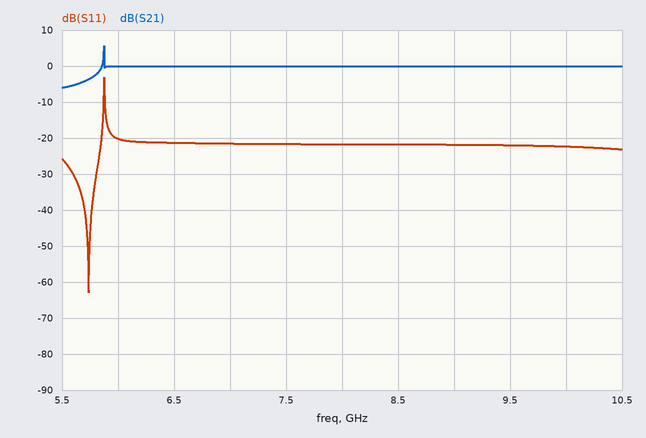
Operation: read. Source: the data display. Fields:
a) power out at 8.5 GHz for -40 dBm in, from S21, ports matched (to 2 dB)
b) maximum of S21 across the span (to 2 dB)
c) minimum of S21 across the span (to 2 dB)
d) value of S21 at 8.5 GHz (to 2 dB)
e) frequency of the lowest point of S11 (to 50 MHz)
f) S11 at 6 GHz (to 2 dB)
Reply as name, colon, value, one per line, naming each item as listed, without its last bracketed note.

power out at 8.5 GHz for -40 dBm in, from S21, ports matched: -40 dBm
maximum of S21 across the span: 6 dB
minimum of S21 across the span: -6 dB
value of S21 at 8.5 GHz: 0 dB
frequency of the lowest point of S11: 5.75 GHz
S11 at 6 GHz: -20 dB
